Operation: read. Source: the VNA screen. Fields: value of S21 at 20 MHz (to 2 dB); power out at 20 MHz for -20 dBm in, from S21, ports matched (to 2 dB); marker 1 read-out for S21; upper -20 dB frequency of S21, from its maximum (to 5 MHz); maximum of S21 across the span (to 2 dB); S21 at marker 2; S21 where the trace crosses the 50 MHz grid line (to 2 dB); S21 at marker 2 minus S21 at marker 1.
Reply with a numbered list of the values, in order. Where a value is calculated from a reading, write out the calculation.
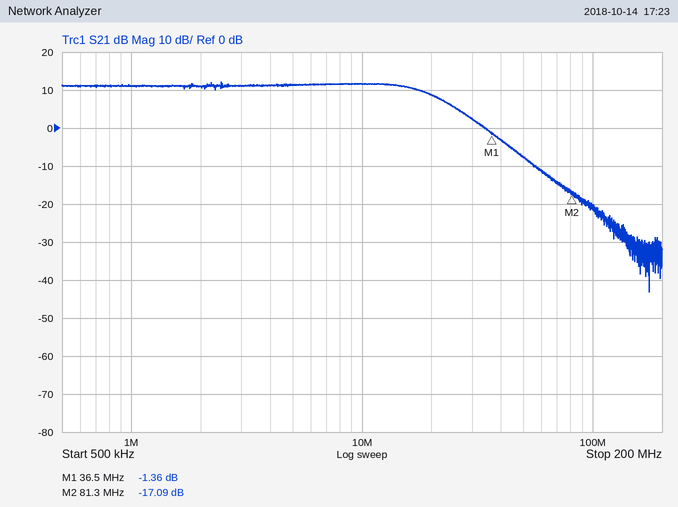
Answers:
1. 8 dB
2. -20 dBm + (8 dB) = -12 dBm
3. -1.36 dB
4. 50 MHz
5. 12 dB
6. -17.09 dB
7. -8 dB
8. -17.09 − (-1.36) = -15.73 dB
